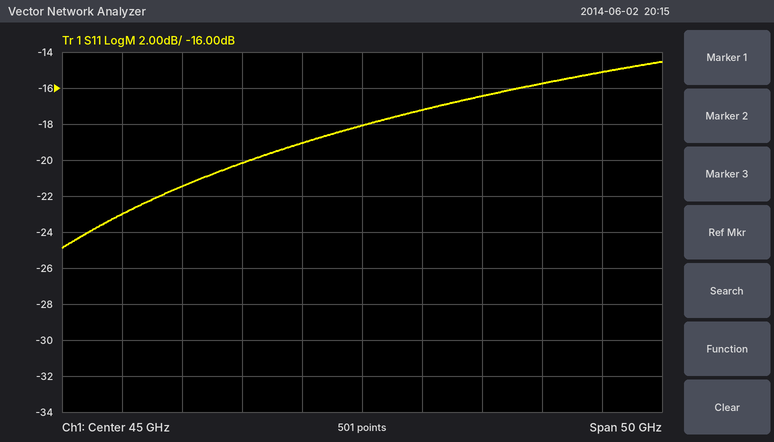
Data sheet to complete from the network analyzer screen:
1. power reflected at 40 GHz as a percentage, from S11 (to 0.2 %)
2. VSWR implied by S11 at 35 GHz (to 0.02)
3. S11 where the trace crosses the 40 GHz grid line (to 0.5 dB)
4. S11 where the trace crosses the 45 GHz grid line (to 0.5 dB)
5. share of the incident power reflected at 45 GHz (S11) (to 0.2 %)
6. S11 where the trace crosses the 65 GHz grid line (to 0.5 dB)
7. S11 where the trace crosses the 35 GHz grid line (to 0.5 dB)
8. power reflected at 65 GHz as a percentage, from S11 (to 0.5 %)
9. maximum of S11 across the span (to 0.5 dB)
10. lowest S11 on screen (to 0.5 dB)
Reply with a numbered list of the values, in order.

1. 1.2 %
2. 1.22
3. -19.0 dB
4. -18.0 dB
5. 1.6 %
6. -15.0 dB
7. -20.0 dB
8. 3.0 %
9. -14.5 dB
10. -25.0 dB
